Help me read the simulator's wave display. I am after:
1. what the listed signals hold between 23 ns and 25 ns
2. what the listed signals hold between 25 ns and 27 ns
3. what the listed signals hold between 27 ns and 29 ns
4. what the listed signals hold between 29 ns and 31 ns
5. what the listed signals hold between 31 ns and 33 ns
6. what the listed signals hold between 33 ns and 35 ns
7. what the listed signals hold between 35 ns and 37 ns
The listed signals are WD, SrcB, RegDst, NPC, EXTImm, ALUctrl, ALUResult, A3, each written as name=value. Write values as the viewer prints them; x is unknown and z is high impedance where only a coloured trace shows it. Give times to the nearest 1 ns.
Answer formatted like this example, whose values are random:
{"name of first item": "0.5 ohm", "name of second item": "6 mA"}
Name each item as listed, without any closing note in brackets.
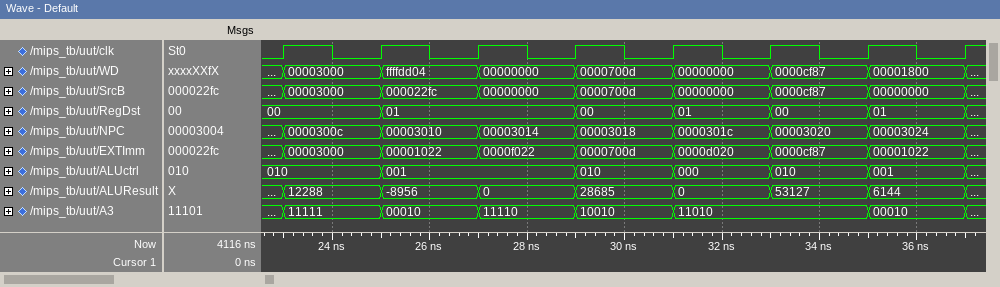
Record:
{"what the listed signals hold between 23 ns and 25 ns": "WD=00003000, SrcB=00003000, RegDst=00, NPC=0000300c, EXTImm=00003000, ALUctrl=010, ALUResult=12288, A3=11111", "what the listed signals hold between 25 ns and 27 ns": "WD=ffffdd04, SrcB=000022fc, RegDst=01, NPC=00003010, EXTImm=00001022, ALUctrl=001, ALUResult=-8956, A3=00010", "what the listed signals hold between 27 ns and 29 ns": "WD=00000000, SrcB=00000000, RegDst=01, NPC=00003014, EXTImm=0000f022, ALUctrl=001, ALUResult=0, A3=11110", "what the listed signals hold between 29 ns and 31 ns": "WD=0000700d, SrcB=0000700d, RegDst=00, NPC=00003018, EXTImm=0000700d, ALUctrl=010, ALUResult=28685, A3=10010", "what the listed signals hold between 31 ns and 33 ns": "WD=00000000, SrcB=00000000, RegDst=01, NPC=0000301c, EXTImm=0000d020, ALUctrl=000, ALUResult=0, A3=11010", "what the listed signals hold between 33 ns and 35 ns": "WD=0000cf87, SrcB=0000cf87, RegDst=00, NPC=00003020, EXTImm=0000cf87, ALUctrl=010, ALUResult=53127, A3=11010", "what the listed signals hold between 35 ns and 37 ns": "WD=00001800, SrcB=00000000, RegDst=01, NPC=00003024, EXTImm=00001022, ALUctrl=001, ALUResult=6144, A3=00010"}
